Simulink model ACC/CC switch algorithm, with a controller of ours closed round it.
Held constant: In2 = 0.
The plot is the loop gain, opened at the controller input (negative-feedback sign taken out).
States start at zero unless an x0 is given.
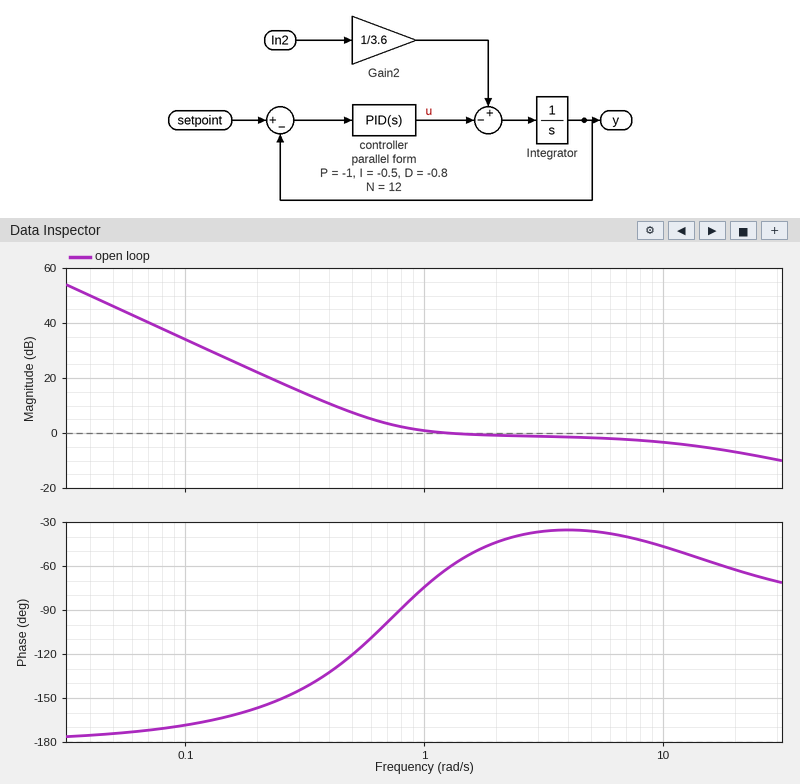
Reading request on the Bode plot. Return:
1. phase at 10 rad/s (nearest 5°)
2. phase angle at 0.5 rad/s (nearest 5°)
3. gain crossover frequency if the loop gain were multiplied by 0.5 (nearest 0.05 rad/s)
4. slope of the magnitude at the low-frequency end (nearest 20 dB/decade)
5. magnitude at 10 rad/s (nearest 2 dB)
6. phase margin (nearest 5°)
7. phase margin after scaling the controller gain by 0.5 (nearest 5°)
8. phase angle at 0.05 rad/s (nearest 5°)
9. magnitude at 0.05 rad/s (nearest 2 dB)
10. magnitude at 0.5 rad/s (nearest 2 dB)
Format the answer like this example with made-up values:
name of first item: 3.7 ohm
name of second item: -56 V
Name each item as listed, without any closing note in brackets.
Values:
phase at 10 rad/s: -45°
phase angle at 0.5 rad/s: -120°
gain crossover frequency if the loop gain were multiplied by 0.5: 0.55 rad/s
slope of the magnitude at the low-frequency end: -40 dB/decade
magnitude at 10 rad/s: -4 dB
phase margin: 120°
phase margin after scaling the controller gain by 0.5: 65°
phase angle at 0.05 rad/s: -175°
magnitude at 0.05 rad/s: 46 dB
magnitude at 0.5 rad/s: 8 dB
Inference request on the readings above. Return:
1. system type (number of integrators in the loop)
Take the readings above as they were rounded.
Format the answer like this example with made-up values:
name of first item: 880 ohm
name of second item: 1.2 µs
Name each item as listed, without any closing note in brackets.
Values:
system type: 2
